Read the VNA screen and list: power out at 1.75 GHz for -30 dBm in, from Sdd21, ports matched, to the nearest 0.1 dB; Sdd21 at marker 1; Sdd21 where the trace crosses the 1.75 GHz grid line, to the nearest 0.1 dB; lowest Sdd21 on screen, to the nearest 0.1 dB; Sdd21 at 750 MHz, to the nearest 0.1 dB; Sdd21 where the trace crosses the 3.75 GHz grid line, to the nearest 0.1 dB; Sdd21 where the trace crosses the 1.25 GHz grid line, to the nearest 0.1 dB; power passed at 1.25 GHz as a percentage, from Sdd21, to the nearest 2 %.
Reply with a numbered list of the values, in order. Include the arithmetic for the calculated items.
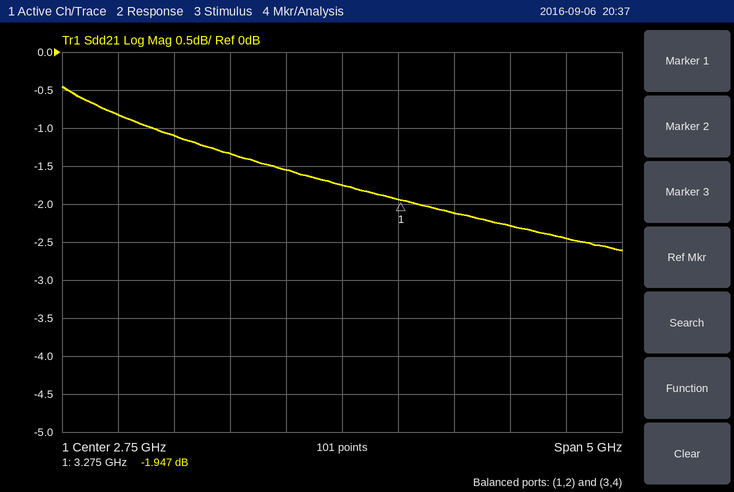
1. -30 dBm + (-1.3 dB) = -31.3 dBm
2. -1.947 dB
3. -1.3 dB
4. -2.6 dB
5. -0.8 dB
6. -2.1 dB
7. -1.1 dB
8. 10^(-1.1/10) ≈ 78 %
